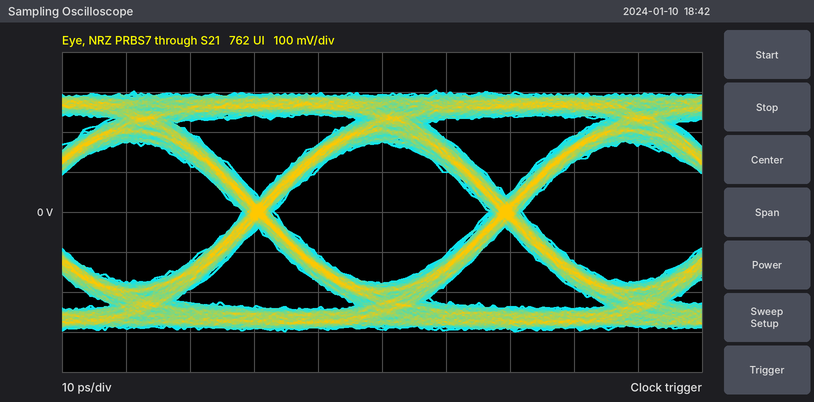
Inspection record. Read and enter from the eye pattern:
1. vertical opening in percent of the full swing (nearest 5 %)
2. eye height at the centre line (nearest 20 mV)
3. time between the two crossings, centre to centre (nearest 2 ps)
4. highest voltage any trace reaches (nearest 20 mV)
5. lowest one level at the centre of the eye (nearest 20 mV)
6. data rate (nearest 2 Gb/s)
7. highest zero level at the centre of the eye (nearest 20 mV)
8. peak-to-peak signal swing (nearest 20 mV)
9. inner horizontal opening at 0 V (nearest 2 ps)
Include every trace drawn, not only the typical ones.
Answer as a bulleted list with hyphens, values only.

- 60 %
- 360 mV
- 38 ps
- 300 mV
- 180 mV
- 26 Gb/s
- -180 mV
- 600 mV
- 34 ps
